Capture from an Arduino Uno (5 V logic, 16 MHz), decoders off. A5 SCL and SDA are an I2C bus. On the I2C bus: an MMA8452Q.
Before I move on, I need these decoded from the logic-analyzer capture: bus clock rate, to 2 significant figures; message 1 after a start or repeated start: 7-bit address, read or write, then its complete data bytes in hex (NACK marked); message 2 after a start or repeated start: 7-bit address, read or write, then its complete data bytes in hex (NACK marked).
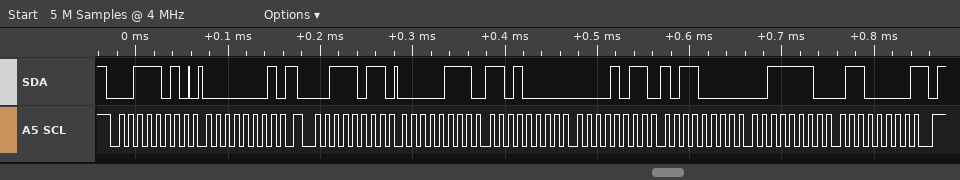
100 kHz
0x1D write: 01
0x1D read: 07 D0 0B B0 3E 60 NACK
